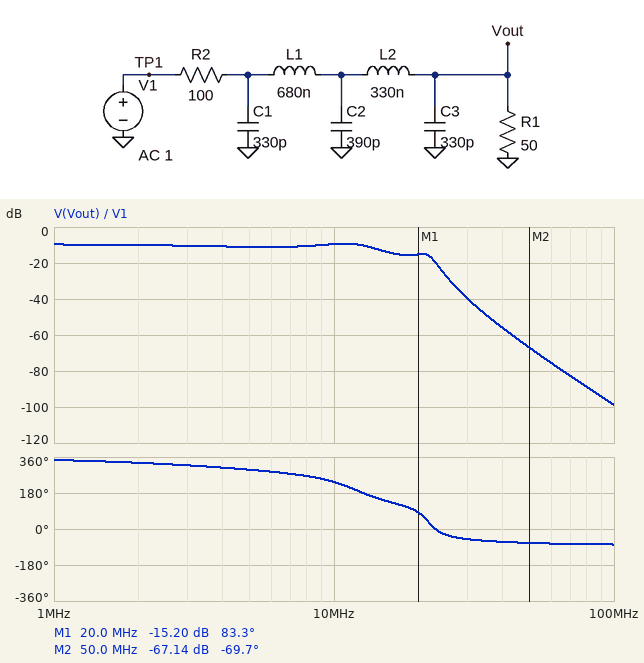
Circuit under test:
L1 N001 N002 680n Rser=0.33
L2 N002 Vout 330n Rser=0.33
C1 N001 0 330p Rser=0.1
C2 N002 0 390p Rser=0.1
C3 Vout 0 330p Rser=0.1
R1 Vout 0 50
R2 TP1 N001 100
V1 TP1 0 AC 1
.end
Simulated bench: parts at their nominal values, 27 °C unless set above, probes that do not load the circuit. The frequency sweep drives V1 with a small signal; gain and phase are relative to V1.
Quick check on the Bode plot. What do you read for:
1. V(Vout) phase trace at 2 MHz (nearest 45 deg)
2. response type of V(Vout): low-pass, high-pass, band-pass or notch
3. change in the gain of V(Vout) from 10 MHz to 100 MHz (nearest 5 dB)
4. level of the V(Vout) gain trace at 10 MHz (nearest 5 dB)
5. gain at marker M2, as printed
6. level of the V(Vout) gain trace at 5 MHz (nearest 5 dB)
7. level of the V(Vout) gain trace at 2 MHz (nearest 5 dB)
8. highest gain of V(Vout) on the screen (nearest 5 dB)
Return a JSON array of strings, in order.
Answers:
["315 deg", "low-pass", "-90 dB", "-10 dB", "-67.14 dB", "-10 dB", "-10 dB", "-10 dB"]
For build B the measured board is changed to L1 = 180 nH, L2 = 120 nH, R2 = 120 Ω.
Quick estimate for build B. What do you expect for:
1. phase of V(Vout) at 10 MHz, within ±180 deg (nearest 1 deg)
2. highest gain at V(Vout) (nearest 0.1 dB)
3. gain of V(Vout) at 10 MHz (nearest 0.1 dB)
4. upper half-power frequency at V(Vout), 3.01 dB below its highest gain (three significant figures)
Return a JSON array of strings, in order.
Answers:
["-77 deg", "-10.6 dB", "-16.2 dB", "25.2 MHz"]
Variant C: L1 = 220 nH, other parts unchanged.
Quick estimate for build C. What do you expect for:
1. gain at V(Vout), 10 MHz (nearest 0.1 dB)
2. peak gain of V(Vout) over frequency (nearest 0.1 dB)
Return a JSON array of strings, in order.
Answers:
["-12.6 dB", "-9.6 dB"]
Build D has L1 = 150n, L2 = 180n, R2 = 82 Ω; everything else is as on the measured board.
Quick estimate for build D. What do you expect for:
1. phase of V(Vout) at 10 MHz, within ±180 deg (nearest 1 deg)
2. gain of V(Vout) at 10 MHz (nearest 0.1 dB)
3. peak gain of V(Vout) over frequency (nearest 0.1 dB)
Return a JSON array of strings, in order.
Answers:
["-78 deg", "-12.9 dB", "-8.5 dB"]
